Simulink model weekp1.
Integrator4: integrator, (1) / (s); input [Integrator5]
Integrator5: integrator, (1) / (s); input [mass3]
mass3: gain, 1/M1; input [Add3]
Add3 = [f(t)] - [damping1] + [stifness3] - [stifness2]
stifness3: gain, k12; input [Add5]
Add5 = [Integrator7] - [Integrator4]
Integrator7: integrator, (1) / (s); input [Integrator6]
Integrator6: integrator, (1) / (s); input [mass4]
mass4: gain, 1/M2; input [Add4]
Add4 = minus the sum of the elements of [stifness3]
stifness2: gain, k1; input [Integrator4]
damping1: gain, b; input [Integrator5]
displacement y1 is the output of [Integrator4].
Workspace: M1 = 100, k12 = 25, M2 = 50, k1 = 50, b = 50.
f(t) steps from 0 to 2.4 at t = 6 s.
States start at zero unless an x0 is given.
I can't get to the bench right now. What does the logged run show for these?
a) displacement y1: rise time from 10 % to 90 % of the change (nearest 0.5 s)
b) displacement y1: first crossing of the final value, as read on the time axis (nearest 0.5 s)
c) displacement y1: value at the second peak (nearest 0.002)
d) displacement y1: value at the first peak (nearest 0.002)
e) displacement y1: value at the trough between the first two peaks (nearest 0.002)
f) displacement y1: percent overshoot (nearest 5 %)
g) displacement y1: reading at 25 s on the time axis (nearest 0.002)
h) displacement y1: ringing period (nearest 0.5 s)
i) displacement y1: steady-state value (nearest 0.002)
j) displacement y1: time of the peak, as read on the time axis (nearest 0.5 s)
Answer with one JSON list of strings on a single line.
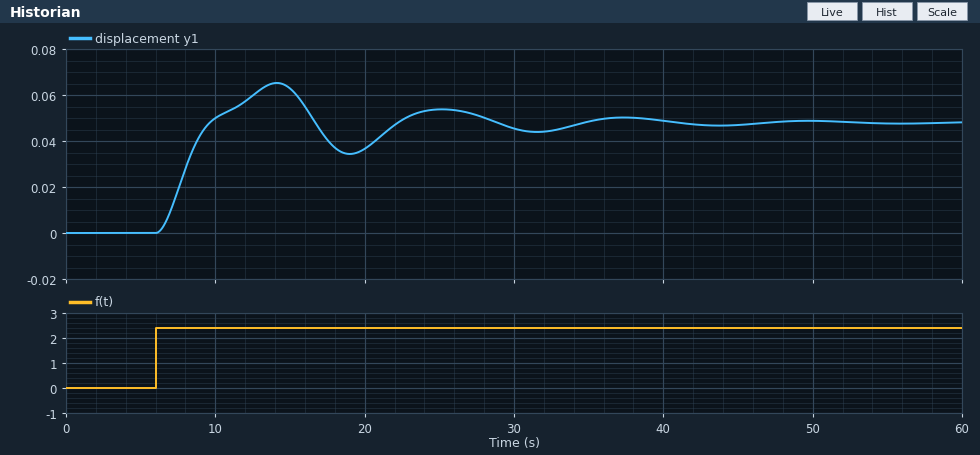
["2.5 s", "9.5 s", "0.054", "0.066", "0.034", "35 %", "0.054", "11.0 s", "0.048", "14.0 s"]
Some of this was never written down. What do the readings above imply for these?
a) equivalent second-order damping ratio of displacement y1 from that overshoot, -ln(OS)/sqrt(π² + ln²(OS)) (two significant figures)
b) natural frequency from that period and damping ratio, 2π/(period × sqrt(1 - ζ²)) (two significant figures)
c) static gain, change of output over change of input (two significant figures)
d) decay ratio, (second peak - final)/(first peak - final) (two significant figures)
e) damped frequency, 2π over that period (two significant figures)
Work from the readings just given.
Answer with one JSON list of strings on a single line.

["0.32", "0.60 rad/s", "0.020", "0.33", "0.57 rad/s"]
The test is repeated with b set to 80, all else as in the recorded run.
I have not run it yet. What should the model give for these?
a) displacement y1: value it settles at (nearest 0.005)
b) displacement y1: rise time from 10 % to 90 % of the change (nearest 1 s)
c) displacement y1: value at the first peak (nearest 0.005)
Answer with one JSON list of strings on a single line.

["0.050", "3 s", "0.060"]
